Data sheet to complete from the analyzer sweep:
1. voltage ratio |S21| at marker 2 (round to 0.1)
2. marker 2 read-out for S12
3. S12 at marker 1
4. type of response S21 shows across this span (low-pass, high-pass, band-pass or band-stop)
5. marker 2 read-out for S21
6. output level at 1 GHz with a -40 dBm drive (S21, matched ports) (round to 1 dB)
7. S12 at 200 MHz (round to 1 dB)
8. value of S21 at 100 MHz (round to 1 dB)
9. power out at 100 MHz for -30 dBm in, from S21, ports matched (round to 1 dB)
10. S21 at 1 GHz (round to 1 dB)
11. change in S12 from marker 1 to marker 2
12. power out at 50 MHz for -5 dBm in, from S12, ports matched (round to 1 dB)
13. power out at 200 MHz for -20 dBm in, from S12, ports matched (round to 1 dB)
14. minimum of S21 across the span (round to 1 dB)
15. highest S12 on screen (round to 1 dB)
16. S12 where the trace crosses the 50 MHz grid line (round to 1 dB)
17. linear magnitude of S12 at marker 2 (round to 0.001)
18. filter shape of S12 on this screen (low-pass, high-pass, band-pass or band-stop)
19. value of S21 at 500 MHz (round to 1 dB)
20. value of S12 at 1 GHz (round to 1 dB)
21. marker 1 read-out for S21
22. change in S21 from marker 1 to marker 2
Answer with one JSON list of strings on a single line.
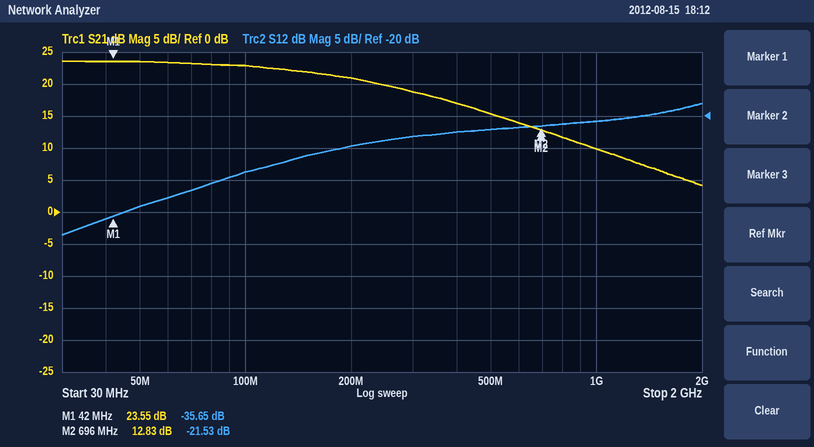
["4.4", "-21.53 dB", "-35.65 dB", "low-pass", "12.83 dB", "-30 dBm", "-25 dB", "23 dB", "-7 dBm", "10 dB", "14.12 dB", "-39 dBm", "-45 dBm", "4 dB", "-18 dB", "-34 dB", "0.084", "high-pass", "15 dB", "-21 dB", "23.55 dB", "-10.72 dB"]
